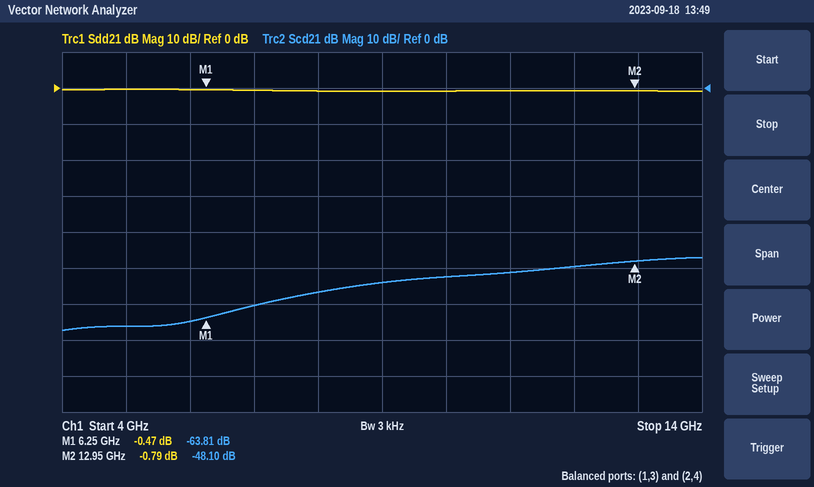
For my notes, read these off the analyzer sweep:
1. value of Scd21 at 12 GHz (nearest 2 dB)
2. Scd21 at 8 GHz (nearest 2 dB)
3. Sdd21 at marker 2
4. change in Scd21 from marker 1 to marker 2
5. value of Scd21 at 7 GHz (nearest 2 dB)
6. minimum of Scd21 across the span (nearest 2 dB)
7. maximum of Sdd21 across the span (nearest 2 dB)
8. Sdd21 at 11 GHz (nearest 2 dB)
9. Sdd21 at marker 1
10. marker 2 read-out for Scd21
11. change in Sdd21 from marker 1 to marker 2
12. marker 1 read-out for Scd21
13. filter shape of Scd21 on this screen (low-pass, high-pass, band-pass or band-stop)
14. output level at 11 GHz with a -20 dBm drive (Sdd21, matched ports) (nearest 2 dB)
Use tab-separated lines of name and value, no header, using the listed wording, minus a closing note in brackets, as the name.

value of Scd21 at 12 GHz	-50 dB
Scd21 at 8 GHz	-56 dB
Sdd21 at marker 2	-0.79 dB
change in Scd21 from marker 1 to marker 2	15.71 dB
value of Scd21 at 7 GHz	-60 dB
minimum of Scd21 across the span	-68 dB
maximum of Sdd21 across the span	0 dB
Sdd21 at 11 GHz	0 dB
Sdd21 at marker 1	-0.47 dB
marker 2 read-out for Scd21	-48.10 dB
change in Sdd21 from marker 1 to marker 2	-0.32 dB
marker 1 read-out for Scd21	-63.81 dB
filter shape of Scd21 on this screen	high-pass
output level at 11 GHz with a -20 dBm drive (Sdd21, matched ports)	-20 dBm
